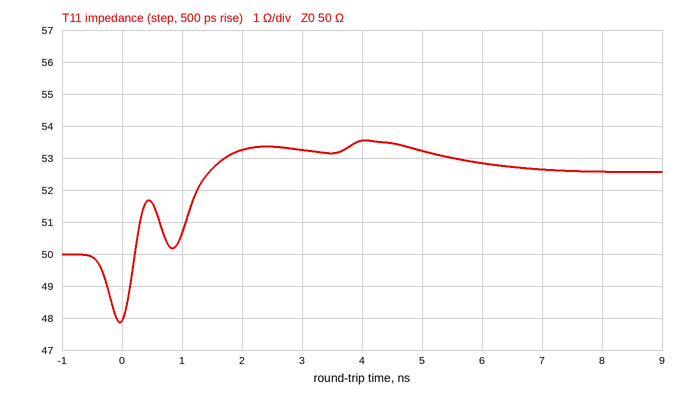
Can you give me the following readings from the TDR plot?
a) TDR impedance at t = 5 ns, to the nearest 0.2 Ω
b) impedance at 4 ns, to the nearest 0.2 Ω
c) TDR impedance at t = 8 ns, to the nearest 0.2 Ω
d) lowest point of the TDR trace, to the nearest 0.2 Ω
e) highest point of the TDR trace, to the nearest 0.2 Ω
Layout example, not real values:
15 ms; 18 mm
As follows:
53.2 Ω; 53.6 Ω; 52.6 Ω; 47.8 Ω; 53.6 Ω
